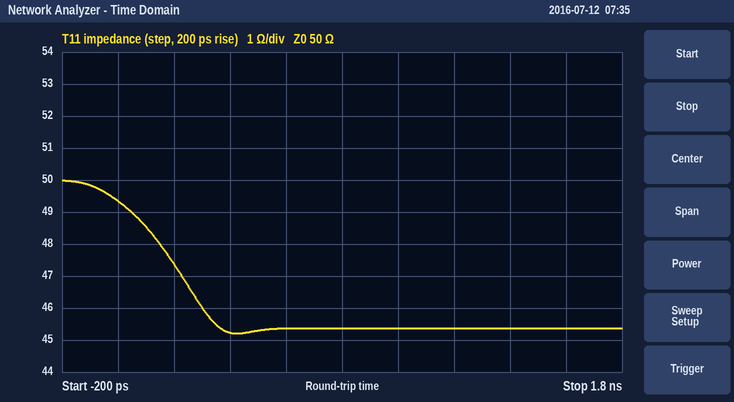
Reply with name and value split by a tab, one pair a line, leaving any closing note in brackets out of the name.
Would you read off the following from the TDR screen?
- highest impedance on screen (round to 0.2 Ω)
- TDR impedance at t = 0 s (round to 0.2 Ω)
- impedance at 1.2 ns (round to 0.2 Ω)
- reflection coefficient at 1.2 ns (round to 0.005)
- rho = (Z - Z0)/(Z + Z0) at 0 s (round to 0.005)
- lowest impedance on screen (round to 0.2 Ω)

highest impedance on screen	50.0 Ω
TDR impedance at t = 0 s	49.4 Ω
impedance at 1.2 ns	45.4 Ω
reflection coefficient at 1.2 ns	-0.050
rho = (Z - Z0)/(Z + Z0) at 0 s	-0.005
lowest impedance on screen	45.2 Ω
